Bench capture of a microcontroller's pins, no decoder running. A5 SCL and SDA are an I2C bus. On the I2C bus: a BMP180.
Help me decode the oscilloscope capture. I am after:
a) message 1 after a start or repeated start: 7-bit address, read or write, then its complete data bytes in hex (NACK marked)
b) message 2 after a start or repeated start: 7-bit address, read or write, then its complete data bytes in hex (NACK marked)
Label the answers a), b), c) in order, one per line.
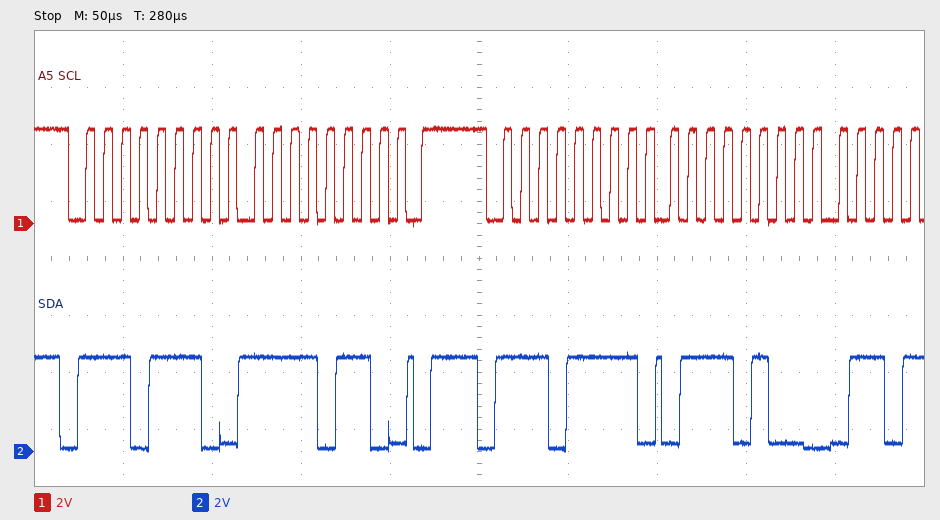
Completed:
a) 0x77 write: F6
b) 0x77 read: 74
